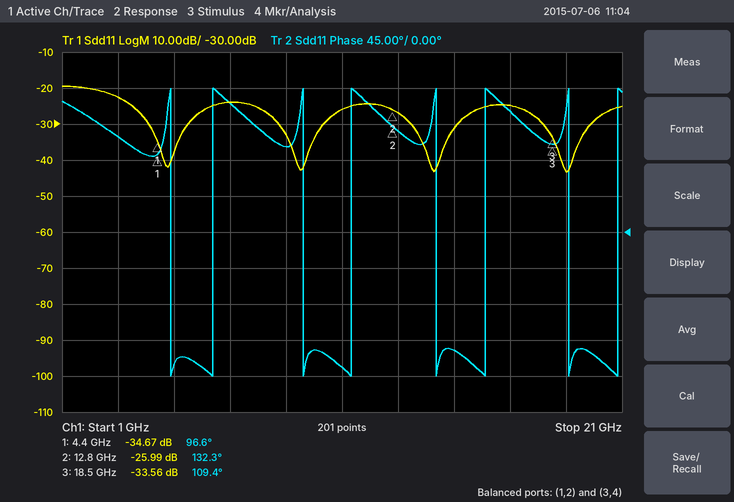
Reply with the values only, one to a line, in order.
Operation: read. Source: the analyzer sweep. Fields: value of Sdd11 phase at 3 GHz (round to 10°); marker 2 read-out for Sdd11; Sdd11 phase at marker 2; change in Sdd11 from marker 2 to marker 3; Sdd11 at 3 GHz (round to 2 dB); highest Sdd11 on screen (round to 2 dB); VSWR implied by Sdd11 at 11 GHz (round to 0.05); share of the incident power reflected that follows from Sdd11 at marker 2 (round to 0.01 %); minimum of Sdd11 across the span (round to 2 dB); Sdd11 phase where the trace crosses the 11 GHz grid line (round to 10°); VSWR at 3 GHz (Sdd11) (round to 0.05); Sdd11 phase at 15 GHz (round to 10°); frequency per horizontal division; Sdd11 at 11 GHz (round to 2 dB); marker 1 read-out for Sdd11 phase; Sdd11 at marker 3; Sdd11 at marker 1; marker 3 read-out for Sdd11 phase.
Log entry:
120°
-25.99 dB
132.3°
-7.57 dB
-22 dB
-20 dB
1.10
0.25 %
-44 dB
-170°
1.15
-150°
2 GHz
-26 dB
96.6°
-33.56 dB
-34.67 dB
109.4°
